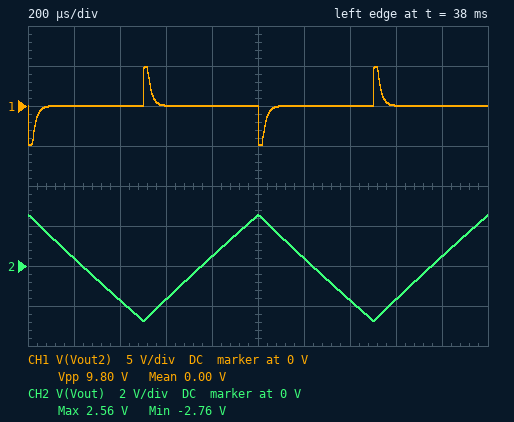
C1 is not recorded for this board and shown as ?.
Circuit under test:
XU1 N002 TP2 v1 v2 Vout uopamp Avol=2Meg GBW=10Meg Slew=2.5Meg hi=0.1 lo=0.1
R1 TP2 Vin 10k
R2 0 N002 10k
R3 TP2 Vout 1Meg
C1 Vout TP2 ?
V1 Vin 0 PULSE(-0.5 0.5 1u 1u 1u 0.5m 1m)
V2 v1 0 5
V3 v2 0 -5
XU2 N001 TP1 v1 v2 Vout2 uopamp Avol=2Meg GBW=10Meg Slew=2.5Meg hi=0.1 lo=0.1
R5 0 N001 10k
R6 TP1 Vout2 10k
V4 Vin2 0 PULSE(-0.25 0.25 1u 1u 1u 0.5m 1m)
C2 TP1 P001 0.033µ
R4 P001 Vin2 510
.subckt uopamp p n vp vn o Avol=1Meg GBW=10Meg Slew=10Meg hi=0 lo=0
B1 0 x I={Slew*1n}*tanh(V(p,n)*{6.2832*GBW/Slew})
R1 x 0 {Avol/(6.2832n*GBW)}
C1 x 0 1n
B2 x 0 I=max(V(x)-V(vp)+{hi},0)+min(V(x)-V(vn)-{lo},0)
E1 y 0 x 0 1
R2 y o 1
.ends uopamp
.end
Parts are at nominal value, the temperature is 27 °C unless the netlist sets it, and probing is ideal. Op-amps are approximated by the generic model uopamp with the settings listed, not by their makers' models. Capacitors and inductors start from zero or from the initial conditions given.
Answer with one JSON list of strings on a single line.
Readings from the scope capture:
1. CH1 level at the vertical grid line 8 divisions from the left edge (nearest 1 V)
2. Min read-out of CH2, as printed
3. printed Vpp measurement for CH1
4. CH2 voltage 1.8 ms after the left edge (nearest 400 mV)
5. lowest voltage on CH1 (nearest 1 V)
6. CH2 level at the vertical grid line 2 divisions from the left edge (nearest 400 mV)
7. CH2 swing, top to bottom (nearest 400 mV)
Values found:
["0 V", "-2.76 V", "9.80 V", "400 mV", "-5 V", "-1.6 V", "5.2 V"]
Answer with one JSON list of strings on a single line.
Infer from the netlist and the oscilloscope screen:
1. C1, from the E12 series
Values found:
["4.7 nF"]
